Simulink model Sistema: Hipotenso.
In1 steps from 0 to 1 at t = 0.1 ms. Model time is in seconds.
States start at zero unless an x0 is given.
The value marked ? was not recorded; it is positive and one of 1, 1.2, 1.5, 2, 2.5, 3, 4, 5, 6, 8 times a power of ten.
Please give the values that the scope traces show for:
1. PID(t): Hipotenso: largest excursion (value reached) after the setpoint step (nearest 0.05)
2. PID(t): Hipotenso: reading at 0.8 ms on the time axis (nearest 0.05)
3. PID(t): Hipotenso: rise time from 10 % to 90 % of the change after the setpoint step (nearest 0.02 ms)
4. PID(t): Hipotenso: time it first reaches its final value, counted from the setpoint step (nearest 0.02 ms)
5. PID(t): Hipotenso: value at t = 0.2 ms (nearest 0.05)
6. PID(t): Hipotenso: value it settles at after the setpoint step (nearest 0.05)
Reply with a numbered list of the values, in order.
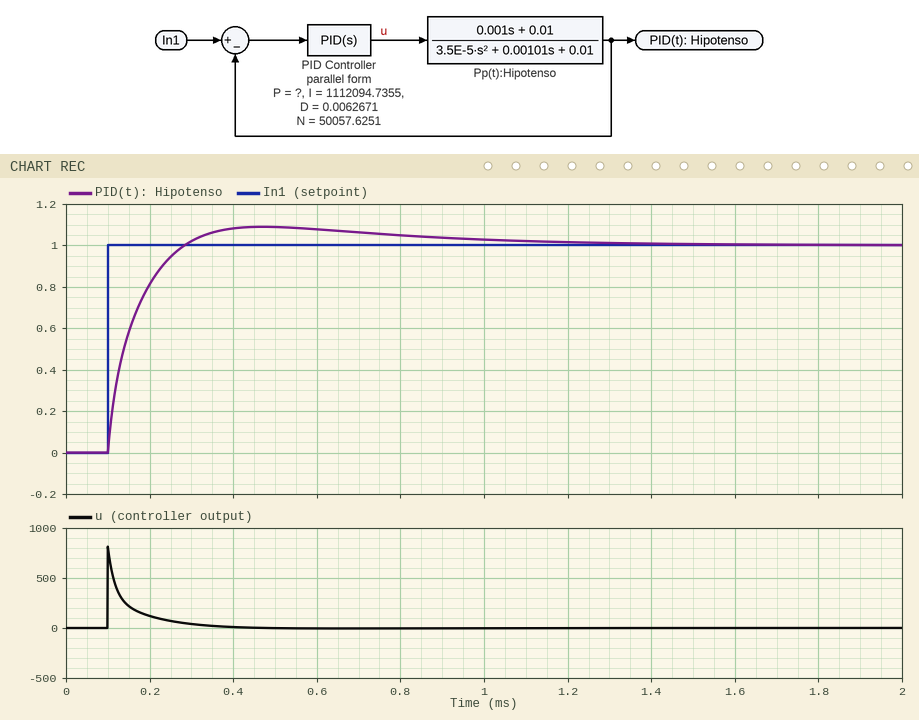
1. 1.10
2. 1.05
3. 0.12 ms
4. 0.18 ms
5. 0.80
6. 1.00
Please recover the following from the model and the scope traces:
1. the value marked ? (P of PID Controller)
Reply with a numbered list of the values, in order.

1. 500
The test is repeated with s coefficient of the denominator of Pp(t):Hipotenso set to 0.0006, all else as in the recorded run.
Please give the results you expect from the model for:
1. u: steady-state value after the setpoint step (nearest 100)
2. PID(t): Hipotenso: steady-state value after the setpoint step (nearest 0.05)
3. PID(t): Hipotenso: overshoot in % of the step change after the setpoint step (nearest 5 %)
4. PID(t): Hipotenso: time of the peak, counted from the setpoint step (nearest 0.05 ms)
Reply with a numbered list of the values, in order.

1. 0
2. 1.00
3. 10 %
4. 0.35 ms
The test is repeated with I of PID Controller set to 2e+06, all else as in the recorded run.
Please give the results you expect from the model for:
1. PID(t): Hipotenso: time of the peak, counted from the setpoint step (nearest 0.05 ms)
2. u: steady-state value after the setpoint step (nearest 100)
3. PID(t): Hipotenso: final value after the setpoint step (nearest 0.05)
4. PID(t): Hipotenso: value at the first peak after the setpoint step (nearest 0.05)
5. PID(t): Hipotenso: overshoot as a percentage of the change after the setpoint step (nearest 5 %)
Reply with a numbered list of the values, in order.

1. 0.30 ms
2. 0
3. 1.00
4. 1.15
5. 15 %
